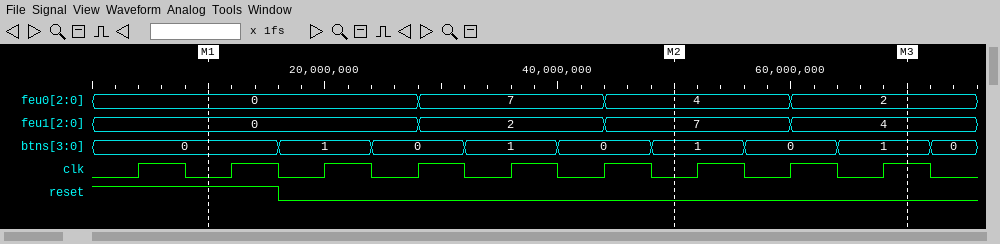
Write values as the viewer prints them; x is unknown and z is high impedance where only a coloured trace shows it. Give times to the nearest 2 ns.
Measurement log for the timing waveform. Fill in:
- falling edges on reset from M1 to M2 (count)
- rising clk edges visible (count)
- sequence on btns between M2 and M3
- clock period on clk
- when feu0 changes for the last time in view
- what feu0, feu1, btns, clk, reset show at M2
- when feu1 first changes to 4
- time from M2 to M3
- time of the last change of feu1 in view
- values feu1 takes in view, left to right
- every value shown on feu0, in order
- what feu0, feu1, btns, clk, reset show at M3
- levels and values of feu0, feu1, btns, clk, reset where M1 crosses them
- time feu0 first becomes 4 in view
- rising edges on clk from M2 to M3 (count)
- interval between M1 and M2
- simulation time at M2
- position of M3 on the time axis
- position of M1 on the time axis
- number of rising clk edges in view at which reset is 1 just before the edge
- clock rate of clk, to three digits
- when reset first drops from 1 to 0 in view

1
9
1, 0, 1
8 ns
60 ns
feu0=4, feu1=7, btns=1, clk=0, reset=0
60 ns
20 ns
60 ns
0, 2, 7, 4
0, 7, 4, 2
feu0=2, feu1=4, btns=1, clk=1, reset=0
feu0=0, feu1=0, btns=0, clk=0, reset=1
44 ns
3
40 ns
50 ns
70 ns
10 ns
2
125 MHz
16 ns
